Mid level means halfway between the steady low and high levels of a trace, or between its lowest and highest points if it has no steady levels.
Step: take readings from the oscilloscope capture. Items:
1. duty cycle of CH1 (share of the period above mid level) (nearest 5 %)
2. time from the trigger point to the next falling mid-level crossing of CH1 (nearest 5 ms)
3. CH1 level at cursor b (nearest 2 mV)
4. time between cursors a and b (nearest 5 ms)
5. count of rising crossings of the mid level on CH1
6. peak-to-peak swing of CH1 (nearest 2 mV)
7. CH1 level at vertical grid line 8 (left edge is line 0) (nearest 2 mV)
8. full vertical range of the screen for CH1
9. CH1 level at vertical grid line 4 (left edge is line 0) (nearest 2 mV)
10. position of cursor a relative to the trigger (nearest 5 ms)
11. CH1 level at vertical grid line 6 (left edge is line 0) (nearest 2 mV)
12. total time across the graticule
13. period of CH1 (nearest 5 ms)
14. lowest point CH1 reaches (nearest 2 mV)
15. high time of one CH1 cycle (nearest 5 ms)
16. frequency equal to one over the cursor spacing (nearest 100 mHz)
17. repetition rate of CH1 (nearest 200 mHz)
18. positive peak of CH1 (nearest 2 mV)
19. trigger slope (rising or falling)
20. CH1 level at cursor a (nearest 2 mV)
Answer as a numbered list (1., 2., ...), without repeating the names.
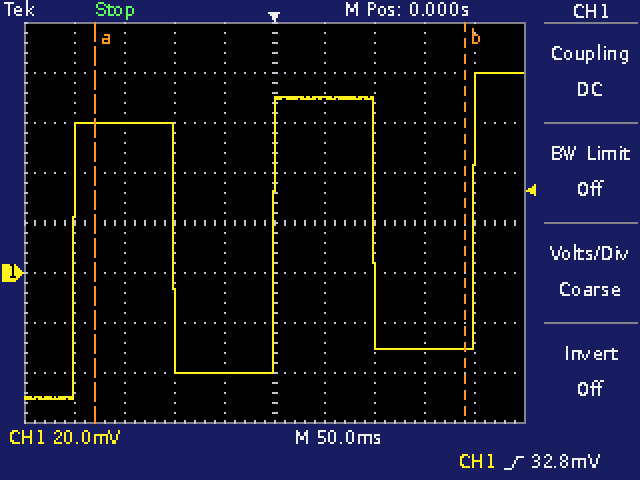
1. 50 %
2. 100 ms
3. -30 mV
4. 370 ms
5. 3
6. 130 mV
7. -30 mV
8. 160 mV
9. -40 mV
10. -180 ms
11. 70 mV
12. 500 ms
13. 200 ms
14. -50 mV
15. 100 ms
16. 2.7 Hz
17. 5.0 Hz
18. 80 mV
19. rising
20. 60 mV
